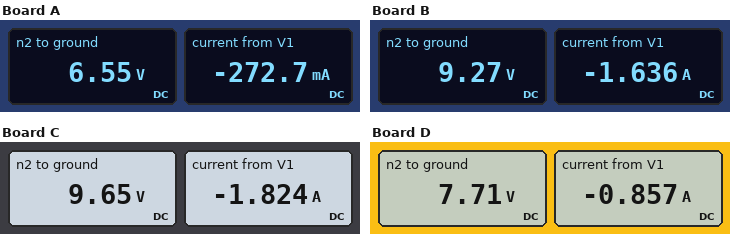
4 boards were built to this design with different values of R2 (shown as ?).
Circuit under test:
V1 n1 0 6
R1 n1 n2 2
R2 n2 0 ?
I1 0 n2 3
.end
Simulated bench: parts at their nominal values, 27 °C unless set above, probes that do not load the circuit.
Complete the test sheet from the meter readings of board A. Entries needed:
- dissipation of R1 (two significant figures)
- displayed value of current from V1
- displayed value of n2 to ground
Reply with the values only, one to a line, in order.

150 mW
-272.7 mA
6.55 V
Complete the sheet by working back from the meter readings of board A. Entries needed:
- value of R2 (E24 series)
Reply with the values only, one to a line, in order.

2.4 Ω
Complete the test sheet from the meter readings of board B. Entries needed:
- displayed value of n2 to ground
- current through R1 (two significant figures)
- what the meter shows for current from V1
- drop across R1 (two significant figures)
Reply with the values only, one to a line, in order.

9.27 V
1.6 A
-1.636 A
3.3 V
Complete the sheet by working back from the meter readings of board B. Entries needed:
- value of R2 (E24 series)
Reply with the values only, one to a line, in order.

6.8 Ω
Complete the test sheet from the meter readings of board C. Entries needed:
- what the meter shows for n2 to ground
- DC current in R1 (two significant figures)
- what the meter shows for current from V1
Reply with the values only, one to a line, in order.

9.65 V
1.8 A
-1.824 A
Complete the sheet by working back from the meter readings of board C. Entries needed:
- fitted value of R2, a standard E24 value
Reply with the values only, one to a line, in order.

8.2 Ω
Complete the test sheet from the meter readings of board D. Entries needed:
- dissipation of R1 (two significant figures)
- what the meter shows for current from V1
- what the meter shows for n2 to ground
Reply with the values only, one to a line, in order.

1.5 W
-0.857 A
7.71 V
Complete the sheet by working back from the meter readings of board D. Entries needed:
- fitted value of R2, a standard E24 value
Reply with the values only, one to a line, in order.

3.6 Ω
